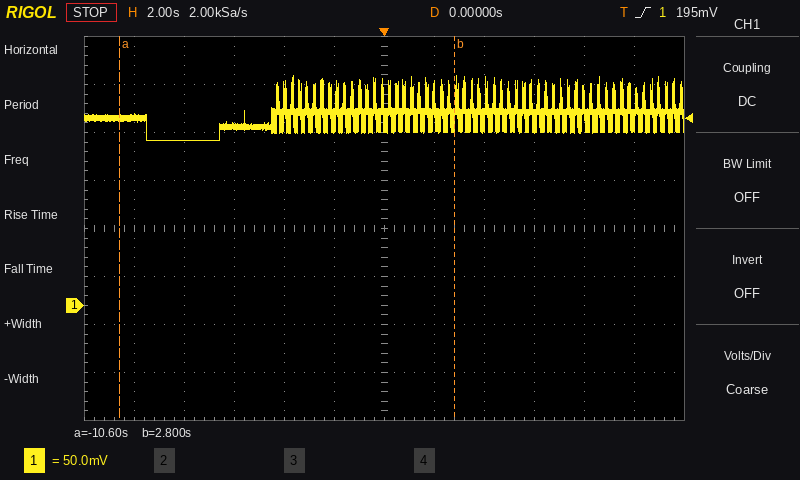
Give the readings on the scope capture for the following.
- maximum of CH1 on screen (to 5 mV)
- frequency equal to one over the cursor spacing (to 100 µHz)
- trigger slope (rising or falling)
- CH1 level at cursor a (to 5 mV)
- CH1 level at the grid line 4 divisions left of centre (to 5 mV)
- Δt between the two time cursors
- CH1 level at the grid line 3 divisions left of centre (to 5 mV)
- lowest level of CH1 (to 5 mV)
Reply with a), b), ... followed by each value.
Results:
a) 240 mV
b) 74.6 mHz
c) rising
d) 195 mV
e) 170 mV
f) 13.4 s
g) 185 mV
h) 170 mV
